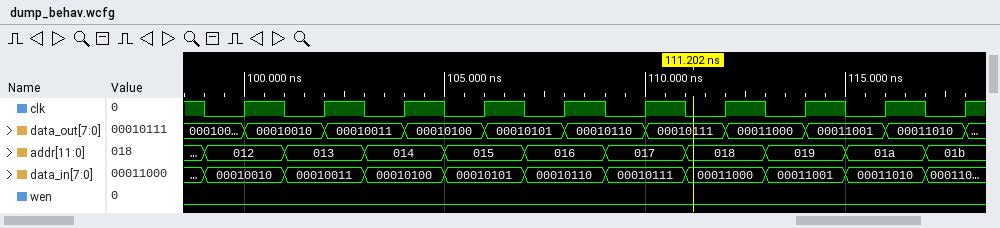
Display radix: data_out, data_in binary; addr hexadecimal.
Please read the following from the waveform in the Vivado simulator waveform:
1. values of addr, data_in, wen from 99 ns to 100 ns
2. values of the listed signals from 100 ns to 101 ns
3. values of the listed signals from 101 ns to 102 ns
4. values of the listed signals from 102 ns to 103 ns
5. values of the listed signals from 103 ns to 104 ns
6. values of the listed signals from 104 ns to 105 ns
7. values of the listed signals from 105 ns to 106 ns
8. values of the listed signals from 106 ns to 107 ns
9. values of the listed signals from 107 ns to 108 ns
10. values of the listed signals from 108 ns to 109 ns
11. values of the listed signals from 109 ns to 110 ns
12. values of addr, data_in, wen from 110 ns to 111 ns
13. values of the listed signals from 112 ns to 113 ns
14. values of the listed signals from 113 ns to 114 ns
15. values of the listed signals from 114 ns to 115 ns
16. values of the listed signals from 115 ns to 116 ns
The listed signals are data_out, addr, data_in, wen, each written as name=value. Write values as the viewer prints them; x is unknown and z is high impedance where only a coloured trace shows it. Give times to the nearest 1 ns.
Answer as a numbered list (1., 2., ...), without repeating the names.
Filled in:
1. addr=012, data_in=00010010, wen=0
2. data_out=00010010, addr=012, data_in=00010010, wen=0
3. data_out=00010010, addr=013, data_in=00010011, wen=0
4. data_out=00010011, addr=013, data_in=00010011, wen=0
5. data_out=00010011, addr=014, data_in=00010100, wen=0
6. data_out=00010100, addr=014, data_in=00010100, wen=0
7. data_out=00010100, addr=015, data_in=00010101, wen=0
8. data_out=00010101, addr=015, data_in=00010101, wen=0
9. data_out=00010101, addr=016, data_in=00010110, wen=0
10. data_out=00010110, addr=016, data_in=00010110, wen=0
11. data_out=00010110, addr=017, data_in=00010111, wen=0
12. addr=017, data_in=00010111, wen=0
13. data_out=00011000, addr=018, data_in=00011000, wen=0
14. data_out=00011000, addr=019, data_in=00011001, wen=0
15. data_out=00011001, addr=019, data_in=00011001, wen=0
16. data_out=00011001, addr=01a, data_in=00011010, wen=0
